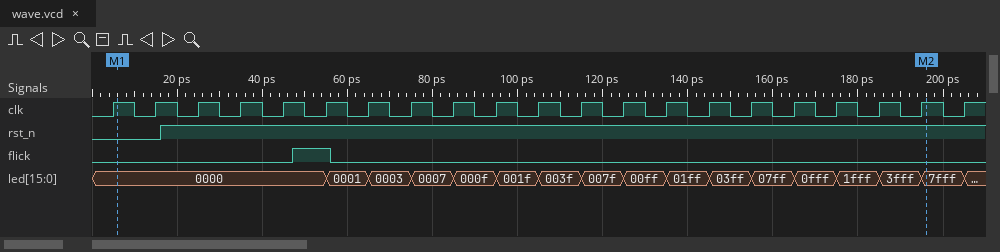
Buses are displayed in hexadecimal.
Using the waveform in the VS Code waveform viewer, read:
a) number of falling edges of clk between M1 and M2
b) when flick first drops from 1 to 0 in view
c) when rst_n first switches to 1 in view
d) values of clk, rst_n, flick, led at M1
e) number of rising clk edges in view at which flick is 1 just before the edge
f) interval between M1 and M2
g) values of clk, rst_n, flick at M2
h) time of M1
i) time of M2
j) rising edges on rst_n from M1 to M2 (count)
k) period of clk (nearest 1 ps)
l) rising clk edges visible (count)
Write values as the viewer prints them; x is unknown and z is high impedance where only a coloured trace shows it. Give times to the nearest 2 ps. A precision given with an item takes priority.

19
56 ps
16 ps
clk=1, rst_n=0, flick=0, led=0000
1
190 ps
clk=1, rst_n=1, flick=0
6 ps
196 ps
1
10 ps
21
